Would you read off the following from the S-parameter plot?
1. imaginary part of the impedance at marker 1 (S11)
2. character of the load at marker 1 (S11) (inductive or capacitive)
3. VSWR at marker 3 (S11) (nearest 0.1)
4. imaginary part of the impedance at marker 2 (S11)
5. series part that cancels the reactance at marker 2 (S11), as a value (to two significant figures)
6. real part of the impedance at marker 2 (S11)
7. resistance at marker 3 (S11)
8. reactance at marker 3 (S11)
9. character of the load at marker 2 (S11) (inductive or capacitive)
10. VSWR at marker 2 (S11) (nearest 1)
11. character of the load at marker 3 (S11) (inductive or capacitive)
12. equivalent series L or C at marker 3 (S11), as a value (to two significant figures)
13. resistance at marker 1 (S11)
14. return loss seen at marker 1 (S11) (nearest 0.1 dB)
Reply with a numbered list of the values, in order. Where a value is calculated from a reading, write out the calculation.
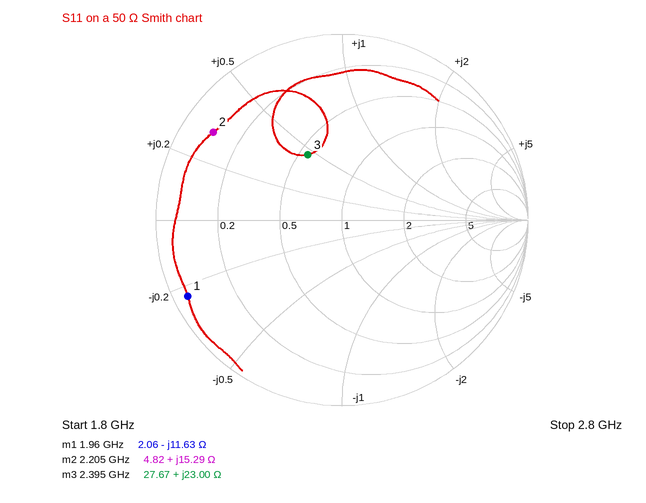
1. -11.63 Ω
2. capacitive
3. 2.3
4. +15.29 Ω
5. C = 1/(2π × 2.205 GHz × 15.29 Ω) ≈ 4.7 pF
6. 4.82 Ω
7. 27.67 Ω
8. +23.00 Ω
9. inductive
10. 11
11. inductive
12. L = 23 Ω/(2π × 2.395 GHz) ≈ 1.5 nH
13. 2.06 Ω
14. 0.7 dB
